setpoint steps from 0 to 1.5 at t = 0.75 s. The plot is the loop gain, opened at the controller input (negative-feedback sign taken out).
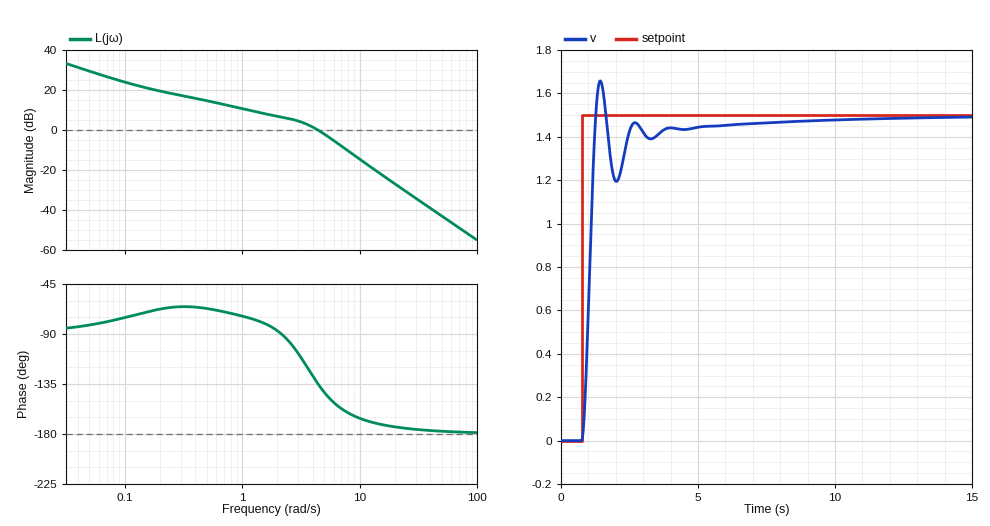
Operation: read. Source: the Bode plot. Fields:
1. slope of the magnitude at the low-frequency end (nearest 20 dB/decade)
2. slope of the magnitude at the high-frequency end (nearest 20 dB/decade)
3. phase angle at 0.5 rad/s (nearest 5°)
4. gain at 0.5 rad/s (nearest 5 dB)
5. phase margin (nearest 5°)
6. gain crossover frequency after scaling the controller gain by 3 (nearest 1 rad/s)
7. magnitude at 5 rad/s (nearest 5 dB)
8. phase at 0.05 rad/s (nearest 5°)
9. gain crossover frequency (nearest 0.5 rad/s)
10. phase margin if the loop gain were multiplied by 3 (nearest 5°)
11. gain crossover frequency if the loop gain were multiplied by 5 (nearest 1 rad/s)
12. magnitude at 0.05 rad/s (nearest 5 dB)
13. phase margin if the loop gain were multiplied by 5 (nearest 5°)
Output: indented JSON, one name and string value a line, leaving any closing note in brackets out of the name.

{
  "slope of the magnitude at the low-frequency end": "-20 dB/decade",
  "slope of the magnitude at the high-frequency end": "-40 dB/decade",
  "phase angle at 0.5 rad/s": "-65°",
  "gain at 0.5 rad/s": "15 dB",
  "phase margin": "45°",
  "gain crossover frequency after scaling the controller gain by 3": "8 rad/s",
  "magnitude at 5 rad/s": "0 dB",
  "phase at 0.05 rad/s": "-80°",
  "gain crossover frequency": "4.5 rad/s",
  "phase margin if the loop gain were multiplied by 3": "20°",
  "gain crossover frequency if the loop gain were multiplied by 5": "10 rad/s",
  "magnitude at 0.05 rad/s": "30 dB",
  "phase margin if the loop gain were multiplied by 5": "15°"
}
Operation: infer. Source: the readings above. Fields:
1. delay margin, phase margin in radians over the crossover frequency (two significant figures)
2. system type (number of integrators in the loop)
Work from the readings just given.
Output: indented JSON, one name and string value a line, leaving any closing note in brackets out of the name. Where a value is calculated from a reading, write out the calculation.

{
  "delay margin, phase margin in radians over the crossover frequency": "45 × π / 180 / 4.5 = 0.17 s",
  "system type": "1"
}
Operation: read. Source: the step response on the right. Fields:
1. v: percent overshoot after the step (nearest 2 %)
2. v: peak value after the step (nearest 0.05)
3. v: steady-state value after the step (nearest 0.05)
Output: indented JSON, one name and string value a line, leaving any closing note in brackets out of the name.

{
  "v: percent overshoot after the step": "10 %",
  "v: peak value after the step": "1.65",
  "v: steady-state value after the step": "1.50"
}
